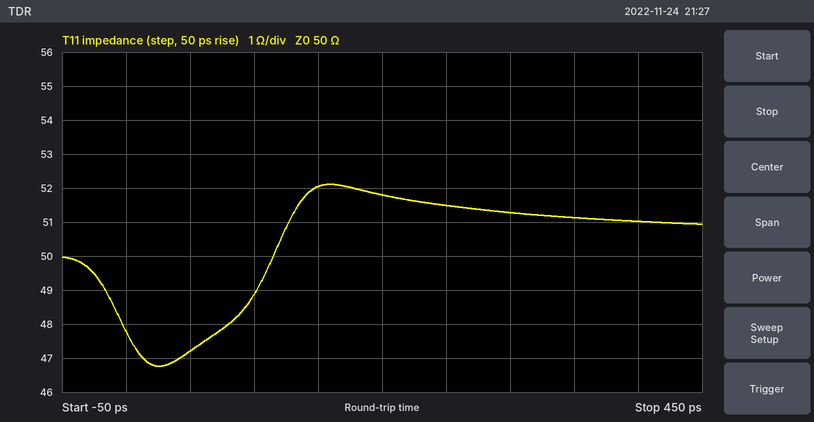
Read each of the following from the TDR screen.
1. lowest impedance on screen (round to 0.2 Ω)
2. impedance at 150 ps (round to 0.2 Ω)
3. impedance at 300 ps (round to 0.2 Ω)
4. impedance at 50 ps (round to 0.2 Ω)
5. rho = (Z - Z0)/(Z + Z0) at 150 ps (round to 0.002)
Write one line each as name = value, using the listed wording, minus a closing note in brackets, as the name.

lowest impedance on screen = 46.8 Ω
impedance at 150 ps = 52.0 Ω
impedance at 300 ps = 51.2 Ω
impedance at 50 ps = 47.2 Ω
rho = (Z - Z0)/(Z + Z0) at 150 ps = +0.020
